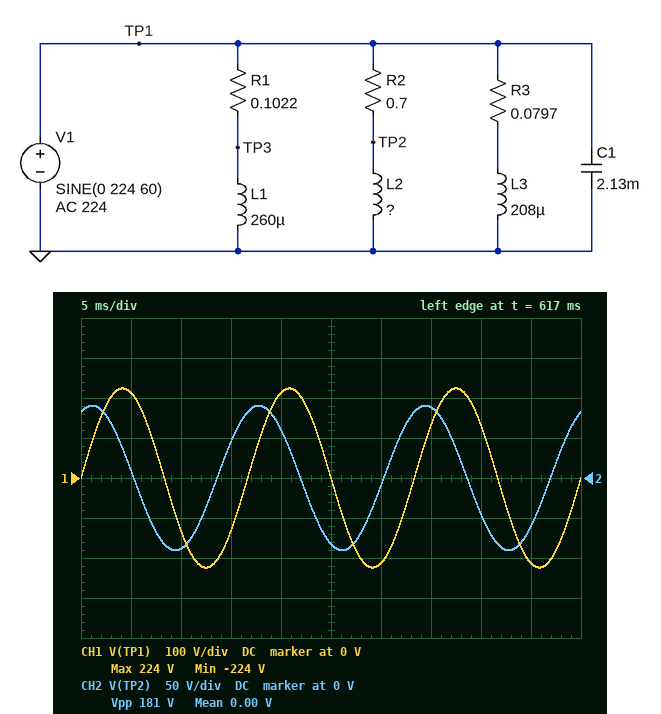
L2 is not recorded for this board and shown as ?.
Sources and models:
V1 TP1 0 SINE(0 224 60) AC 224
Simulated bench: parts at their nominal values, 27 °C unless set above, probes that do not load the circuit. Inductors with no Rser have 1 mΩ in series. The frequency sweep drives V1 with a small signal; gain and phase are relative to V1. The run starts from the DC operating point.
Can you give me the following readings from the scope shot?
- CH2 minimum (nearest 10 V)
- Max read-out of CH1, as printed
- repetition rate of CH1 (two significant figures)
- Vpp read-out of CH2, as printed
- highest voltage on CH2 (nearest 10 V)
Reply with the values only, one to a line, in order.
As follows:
-90 V
224 V
60 Hz
181 V
90 V
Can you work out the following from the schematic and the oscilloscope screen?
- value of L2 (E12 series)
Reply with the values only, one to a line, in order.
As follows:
820 µH
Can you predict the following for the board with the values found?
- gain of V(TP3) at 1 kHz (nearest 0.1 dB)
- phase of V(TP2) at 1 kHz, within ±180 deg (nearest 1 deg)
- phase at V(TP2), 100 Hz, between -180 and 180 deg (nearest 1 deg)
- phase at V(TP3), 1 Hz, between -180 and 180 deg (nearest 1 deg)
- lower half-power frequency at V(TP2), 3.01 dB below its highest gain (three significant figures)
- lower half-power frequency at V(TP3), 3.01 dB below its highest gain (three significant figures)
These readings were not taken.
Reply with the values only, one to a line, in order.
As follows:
0 dB
8 deg
54 deg
58 deg
136 Hz
63.2 Hz
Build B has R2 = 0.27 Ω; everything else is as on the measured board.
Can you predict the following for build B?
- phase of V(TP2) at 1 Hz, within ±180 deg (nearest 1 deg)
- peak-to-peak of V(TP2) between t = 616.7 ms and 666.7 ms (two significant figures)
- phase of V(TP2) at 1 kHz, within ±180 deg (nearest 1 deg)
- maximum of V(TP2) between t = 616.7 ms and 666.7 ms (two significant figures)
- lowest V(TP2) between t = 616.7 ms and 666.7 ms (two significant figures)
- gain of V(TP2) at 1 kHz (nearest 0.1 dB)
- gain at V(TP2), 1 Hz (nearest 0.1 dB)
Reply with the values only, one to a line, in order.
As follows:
78 deg
340 V
3 deg
170 V
-170 V
0 dB
-34.3 dB
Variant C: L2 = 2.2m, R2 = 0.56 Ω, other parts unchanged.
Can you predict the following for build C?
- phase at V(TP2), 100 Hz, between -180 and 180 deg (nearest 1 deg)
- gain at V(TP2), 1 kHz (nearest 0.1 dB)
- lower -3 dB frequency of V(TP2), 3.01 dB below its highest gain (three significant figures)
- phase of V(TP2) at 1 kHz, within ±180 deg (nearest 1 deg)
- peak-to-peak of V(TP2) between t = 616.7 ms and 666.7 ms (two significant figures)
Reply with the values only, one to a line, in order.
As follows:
22 deg
0 dB
40.6 Hz
2 deg
370 V
